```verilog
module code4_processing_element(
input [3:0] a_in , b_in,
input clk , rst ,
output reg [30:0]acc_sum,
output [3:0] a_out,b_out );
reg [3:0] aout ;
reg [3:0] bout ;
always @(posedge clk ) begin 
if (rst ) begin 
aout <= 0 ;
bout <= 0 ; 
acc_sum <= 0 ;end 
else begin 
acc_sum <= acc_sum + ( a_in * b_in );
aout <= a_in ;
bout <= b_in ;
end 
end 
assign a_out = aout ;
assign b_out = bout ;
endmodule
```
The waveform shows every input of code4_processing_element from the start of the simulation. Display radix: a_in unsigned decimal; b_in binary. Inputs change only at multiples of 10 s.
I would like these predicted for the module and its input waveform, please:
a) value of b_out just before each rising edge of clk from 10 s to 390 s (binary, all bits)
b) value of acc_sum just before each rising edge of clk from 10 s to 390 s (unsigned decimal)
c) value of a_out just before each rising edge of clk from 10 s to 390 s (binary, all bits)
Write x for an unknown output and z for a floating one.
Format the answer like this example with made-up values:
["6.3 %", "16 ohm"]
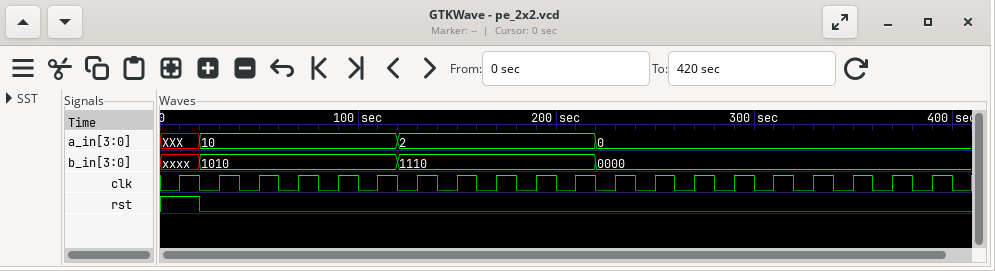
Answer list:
["x, 0000, 1010, 1010, 1010, 1010, 1010, 1110, 1110, 1110, 1110, 1110, 0000, 0000, 0000, 0000, 0000, 0000, 0000, 0000", "x, 0, 100, 200, 300, 400, 500, 528, 556, 584, 612, 640, 640, 640, 640, 640, 640, 640, 640, 640", "x, 0000, 1010, 1010, 1010, 1010, 1010, 0010, 0010, 0010, 0010, 0010, 0000, 0000, 0000, 0000, 0000, 0000, 0000, 0000"]
